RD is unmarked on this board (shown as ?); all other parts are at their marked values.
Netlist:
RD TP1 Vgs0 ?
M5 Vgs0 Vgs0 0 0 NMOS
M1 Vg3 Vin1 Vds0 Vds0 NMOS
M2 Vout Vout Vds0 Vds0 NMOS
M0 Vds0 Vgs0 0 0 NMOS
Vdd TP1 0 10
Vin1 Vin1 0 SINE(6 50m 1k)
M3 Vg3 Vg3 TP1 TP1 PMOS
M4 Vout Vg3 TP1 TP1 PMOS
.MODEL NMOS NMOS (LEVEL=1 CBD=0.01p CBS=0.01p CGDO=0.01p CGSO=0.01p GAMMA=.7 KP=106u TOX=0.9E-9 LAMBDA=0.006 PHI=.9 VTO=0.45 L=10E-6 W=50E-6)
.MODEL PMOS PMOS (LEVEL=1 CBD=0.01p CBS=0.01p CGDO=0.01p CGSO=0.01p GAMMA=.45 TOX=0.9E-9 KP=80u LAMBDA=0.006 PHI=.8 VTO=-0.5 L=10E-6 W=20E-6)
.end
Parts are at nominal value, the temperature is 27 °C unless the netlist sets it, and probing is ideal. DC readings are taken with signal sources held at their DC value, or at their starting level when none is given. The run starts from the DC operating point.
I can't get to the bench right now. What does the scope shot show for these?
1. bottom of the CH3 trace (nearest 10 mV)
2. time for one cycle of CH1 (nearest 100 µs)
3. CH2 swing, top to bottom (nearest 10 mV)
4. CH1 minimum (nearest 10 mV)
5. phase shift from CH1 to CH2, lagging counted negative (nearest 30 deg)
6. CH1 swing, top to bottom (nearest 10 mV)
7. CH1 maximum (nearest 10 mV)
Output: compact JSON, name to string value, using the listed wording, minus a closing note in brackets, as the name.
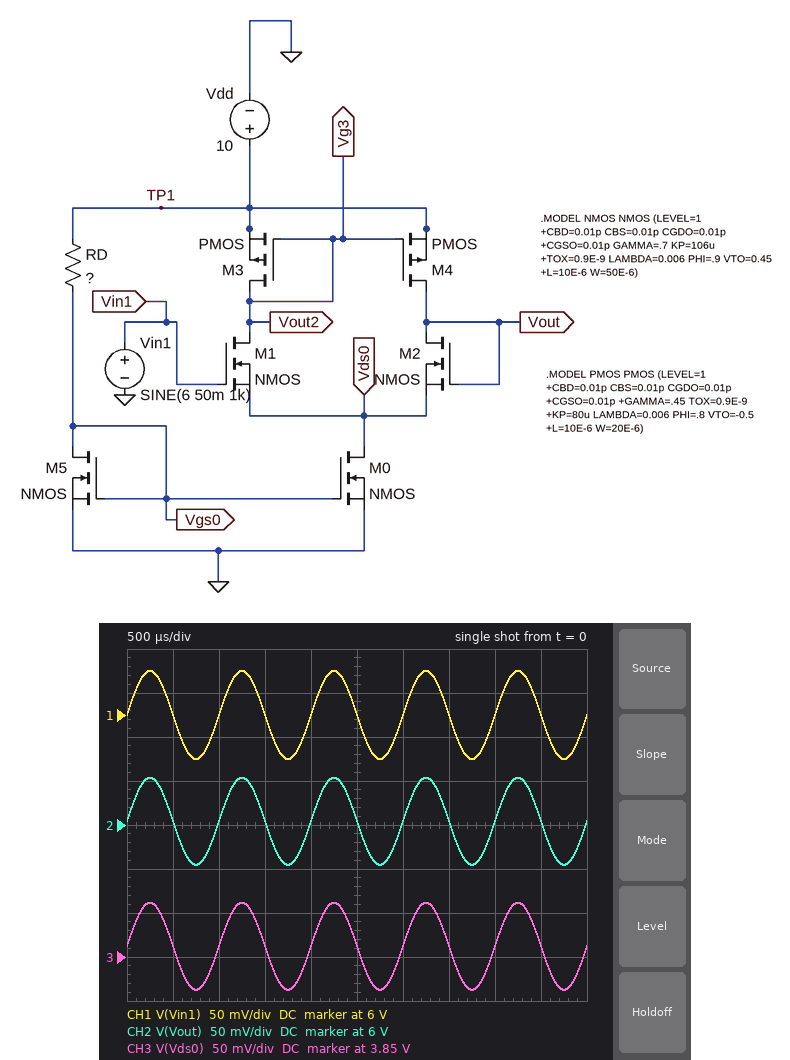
{"bottom of the CH3 trace": "3.81 V", "time for one cycle of CH1": "1.0 ms", "CH2 swing, top to bottom": "100 mV", "CH1 minimum": "5.95 V", "phase shift from CH1 to CH2, lagging counted negative": "0 deg", "CH1 swing, top to bottom": "100 mV", "CH1 maximum": "6.05 V"}
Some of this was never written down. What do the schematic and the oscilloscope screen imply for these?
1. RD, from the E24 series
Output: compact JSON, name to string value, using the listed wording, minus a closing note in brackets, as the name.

{"RD, from the E24 series": "4.7 kΩ"}
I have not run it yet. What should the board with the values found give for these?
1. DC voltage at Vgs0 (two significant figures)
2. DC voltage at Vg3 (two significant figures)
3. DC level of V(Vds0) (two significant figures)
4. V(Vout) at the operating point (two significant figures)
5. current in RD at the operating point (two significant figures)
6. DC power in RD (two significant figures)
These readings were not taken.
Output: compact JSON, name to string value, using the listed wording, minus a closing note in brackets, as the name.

{"DC voltage at Vgs0": "2.8 V", "DC voltage at Vg3": "6.4 V", "DC level of V(Vds0)": "3.9 V", "V(Vout) at the operating point": "6.0 V", "current in RD at the operating point": "1.5 mA", "DC power in RD": "11 mW"}
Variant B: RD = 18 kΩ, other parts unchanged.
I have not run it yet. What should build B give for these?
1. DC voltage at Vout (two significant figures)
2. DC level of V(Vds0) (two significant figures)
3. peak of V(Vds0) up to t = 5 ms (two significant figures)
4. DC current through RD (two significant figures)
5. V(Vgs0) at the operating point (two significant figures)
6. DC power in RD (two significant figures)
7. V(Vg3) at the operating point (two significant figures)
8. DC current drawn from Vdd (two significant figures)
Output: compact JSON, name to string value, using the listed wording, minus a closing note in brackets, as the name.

{"DC voltage at Vout": "6.0 V", "DC level of V(Vds0)": "4.6 V", "peak of V(Vds0) up to t = 5 ms": "4.7 V", "DC current through RD": "460 µA", "V(Vgs0) at the operating point": "1.8 V", "DC power in RD": "3.8 mW", "V(Vg3) at the operating point": "7.8 V", "DC current drawn from Vdd": "920 µA"}
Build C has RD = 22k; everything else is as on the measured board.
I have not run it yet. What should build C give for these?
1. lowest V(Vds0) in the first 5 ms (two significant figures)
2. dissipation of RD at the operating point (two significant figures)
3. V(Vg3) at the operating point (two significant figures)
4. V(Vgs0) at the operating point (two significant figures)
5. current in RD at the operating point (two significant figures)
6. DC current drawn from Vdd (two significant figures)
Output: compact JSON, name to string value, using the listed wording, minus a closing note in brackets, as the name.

{"lowest V(Vds0) in the first 5 ms": "4.7 V", "dissipation of RD at the operating point": "3.2 mW", "V(Vg3) at the operating point": "8.0 V", "V(Vgs0) at the operating point": "1.6 V", "current in RD at the operating point": "380 µA", "DC current drawn from Vdd": "770 µA"}
